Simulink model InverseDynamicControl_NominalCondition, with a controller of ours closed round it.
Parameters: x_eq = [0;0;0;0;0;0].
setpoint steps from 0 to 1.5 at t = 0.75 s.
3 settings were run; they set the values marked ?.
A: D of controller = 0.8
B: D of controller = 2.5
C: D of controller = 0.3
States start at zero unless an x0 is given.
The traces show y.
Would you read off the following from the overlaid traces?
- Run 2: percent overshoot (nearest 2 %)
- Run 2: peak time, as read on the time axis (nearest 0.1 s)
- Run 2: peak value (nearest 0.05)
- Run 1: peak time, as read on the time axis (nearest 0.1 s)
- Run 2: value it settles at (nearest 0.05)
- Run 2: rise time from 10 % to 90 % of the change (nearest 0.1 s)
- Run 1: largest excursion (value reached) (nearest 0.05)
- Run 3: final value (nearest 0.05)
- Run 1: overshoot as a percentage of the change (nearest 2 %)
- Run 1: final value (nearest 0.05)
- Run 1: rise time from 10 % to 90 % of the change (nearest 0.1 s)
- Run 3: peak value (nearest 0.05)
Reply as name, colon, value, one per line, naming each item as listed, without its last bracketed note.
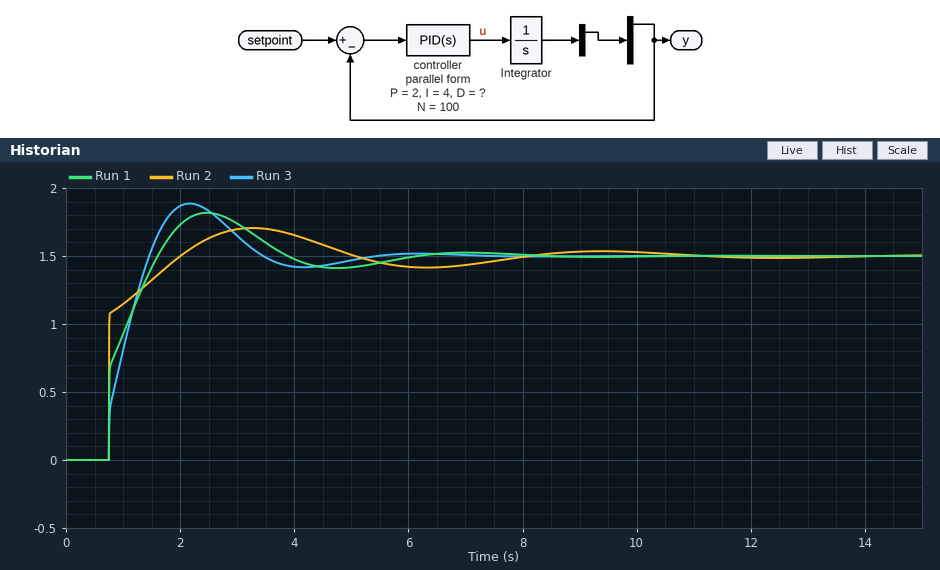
Run 2: percent overshoot: 14 %
Run 2: peak time, as read on the time axis: 3.3 s
Run 2: peak value: 1.70
Run 1: peak time, as read on the time axis: 2.5 s
Run 2: value it settles at: 1.50
Run 2: rise time from 10 % to 90 % of the change: 0.8 s
Run 1: largest excursion (value reached): 1.80
Run 3: final value: 1.50
Run 1: overshoot as a percentage of the change: 22 %
Run 1: final value: 1.50
Run 1: rise time from 10 % to 90 % of the change: 0.7 s
Run 3: peak value: 1.90
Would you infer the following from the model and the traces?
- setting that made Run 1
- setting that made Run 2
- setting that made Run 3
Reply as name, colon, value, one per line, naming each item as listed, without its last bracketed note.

setting that made Run 1: A
setting that made Run 2: B
setting that made Run 3: C
